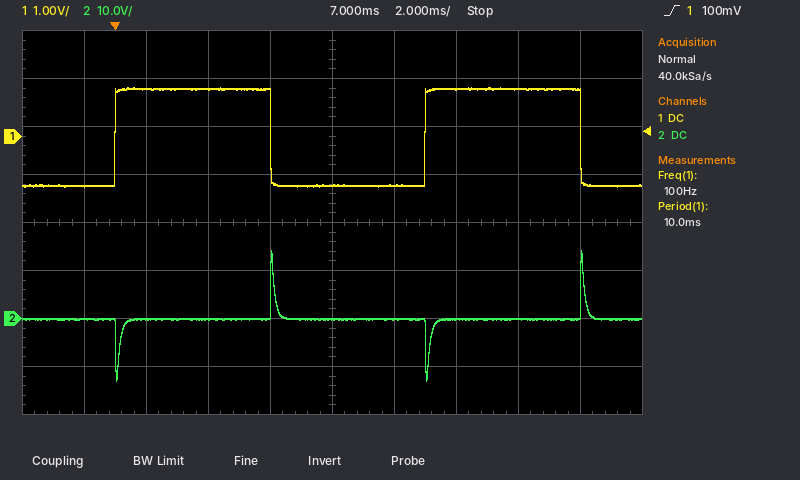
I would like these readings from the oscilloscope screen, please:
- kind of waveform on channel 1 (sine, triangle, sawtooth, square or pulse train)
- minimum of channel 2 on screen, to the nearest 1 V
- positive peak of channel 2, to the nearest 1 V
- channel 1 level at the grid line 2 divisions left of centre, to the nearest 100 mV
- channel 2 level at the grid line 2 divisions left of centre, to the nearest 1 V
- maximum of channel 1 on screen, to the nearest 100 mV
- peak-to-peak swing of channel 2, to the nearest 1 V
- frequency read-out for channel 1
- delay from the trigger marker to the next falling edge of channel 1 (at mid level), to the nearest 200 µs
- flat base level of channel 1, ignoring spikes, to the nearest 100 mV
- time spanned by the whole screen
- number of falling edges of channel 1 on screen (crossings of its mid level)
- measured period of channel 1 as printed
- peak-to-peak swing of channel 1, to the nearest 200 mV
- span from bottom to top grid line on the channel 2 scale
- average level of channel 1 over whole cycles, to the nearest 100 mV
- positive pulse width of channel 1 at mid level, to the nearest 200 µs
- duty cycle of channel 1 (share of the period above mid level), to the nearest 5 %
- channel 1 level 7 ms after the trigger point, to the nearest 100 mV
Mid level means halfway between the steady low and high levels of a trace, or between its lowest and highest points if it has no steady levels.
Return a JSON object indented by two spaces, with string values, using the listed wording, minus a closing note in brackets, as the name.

{
  "kind of waveform on channel 1": "square",
  "minimum of channel 2 on screen, to the nearest 1 V": "-13 V",
  "positive peak of channel 2, to the nearest 1 V": "14 V",
  "channel 1 level at the grid line 2 divisions left of centre, to the nearest 100 mV": "1.0 V",
  "channel 2 level at the grid line 2 divisions left of centre, to the nearest 1 V": "0 V",
  "maximum of channel 1 on screen, to the nearest 100 mV": "1.0 V",
  "peak-to-peak swing of channel 2, to the nearest 1 V": "27 V",
  "frequency read-out for channel 1": "100 Hz",
  "delay from the trigger marker to the next falling edge of channel 1 (at mid level), to the nearest 200 µs": "5.0 ms",
  "flat base level of channel 1, ignoring spikes, to the nearest 100 mV": "-1.0 V",
  "time spanned by the whole screen": "20 ms",
  "number of falling edges of channel 1 on screen": "2",
  "measured period of channel 1 as printed": "10.0 ms",
  "peak-to-peak swing of channel 1, to the nearest 200 mV": "2.0 V",
  "span from bottom to top grid line on the channel 2 scale": "80 V",
  "average level of channel 1 over whole cycles, to the nearest 100 mV": "0.0 V",
  "positive pulse width of channel 1 at mid level, to the nearest 200 µs": "5.0 ms",
  "duty cycle of channel 1 (share of the period above mid level), to the nearest 5 %": "50 %",
  "channel 1 level 7 ms after the trigger point, to the nearest 100 mV": "-1.0 V"
}
